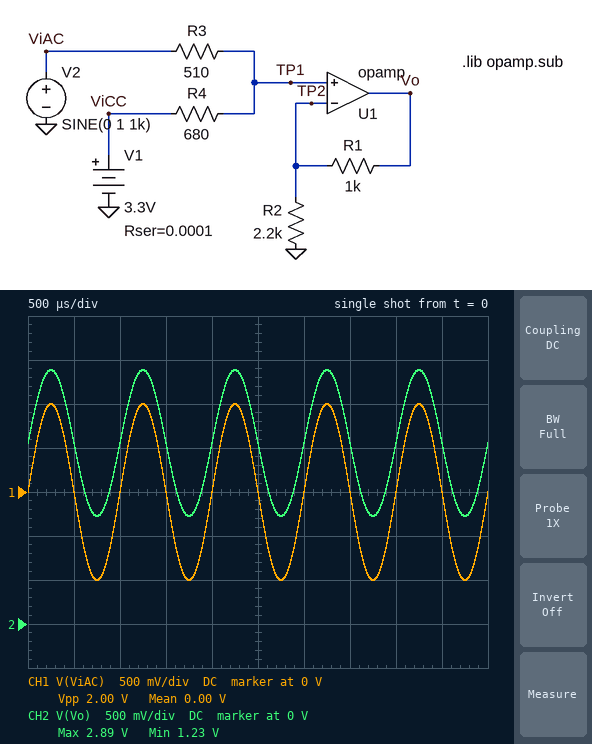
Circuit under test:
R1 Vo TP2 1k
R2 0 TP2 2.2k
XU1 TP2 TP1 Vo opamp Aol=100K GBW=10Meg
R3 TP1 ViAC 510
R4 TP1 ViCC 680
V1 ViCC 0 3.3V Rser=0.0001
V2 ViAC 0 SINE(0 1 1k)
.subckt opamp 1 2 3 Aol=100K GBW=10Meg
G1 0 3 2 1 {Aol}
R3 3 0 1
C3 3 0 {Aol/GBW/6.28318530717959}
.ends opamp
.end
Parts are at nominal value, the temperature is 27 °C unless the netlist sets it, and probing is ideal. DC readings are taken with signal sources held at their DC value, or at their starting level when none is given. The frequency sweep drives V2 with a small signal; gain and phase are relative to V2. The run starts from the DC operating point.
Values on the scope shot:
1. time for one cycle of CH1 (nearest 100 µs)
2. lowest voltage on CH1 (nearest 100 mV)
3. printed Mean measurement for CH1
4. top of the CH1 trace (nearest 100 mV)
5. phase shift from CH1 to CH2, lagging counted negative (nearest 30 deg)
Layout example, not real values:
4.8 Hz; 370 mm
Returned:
1.0 ms; -1.0 V; 0.00 V; 1.0 V; 0 deg
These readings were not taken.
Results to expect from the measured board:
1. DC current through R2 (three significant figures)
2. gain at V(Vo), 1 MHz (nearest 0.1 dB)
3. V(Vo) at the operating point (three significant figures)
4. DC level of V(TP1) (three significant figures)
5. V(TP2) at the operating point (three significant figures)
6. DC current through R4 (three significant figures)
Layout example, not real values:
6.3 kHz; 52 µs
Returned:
643 µA; -1.7 dB; 2.06 V; 1.41 V; 1.41 V; 2.77 mA
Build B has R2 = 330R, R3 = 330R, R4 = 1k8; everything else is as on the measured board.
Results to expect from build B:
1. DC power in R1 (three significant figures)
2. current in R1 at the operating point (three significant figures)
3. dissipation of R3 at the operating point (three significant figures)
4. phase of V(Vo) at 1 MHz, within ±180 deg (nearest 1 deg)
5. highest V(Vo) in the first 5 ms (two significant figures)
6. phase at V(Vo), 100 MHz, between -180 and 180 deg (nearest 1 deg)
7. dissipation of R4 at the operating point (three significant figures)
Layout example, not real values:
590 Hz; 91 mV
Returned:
2.40 mW; 1.55 mA; 792 µW; -22 deg; 5.5 V; -89 deg; 4.32 mW
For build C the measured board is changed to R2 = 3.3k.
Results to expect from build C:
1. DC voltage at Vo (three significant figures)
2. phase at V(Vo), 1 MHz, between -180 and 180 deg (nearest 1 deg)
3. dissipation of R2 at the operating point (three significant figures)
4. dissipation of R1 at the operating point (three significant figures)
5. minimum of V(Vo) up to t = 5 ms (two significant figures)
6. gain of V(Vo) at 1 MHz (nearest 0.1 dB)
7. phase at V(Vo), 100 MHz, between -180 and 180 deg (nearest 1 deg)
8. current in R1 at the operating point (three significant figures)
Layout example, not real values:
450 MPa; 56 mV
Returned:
1.84 V; -7 deg; 606 µW; 184 µW; 1.1 V; -2.6 dB; -86 deg; 429 µA
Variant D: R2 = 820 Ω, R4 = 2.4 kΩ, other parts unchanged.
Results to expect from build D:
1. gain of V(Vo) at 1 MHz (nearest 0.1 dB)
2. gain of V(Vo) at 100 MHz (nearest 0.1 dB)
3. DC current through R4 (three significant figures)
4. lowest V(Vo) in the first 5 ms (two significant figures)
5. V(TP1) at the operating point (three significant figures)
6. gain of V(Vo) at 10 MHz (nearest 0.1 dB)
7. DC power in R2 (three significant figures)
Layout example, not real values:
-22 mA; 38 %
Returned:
5.0 dB; -21.7 dB; 1.13 mA; -550 mV; 578 mV; -2.5 dB; 408 µW
